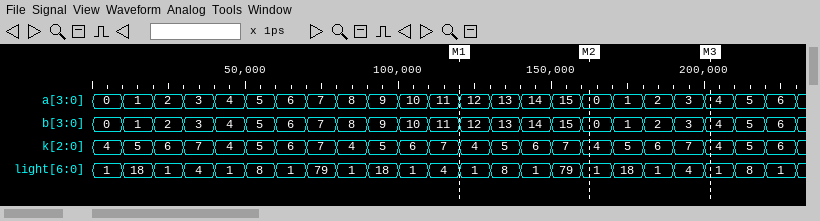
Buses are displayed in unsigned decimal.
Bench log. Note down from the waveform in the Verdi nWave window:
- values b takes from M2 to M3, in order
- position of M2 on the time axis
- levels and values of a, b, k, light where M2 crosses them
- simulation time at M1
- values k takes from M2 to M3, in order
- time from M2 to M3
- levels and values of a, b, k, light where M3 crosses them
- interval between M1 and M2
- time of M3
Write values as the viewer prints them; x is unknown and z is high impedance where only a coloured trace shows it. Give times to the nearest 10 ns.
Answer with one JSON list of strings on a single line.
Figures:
["0, 1, 2, 3, 4", "160 ns", "a=0, b=0, k=4, light=1", "120 ns", "4, 5, 6, 7, 4", "40 ns", "a=4, b=4, k=4, light=1", "40 ns", "200 ns"]
